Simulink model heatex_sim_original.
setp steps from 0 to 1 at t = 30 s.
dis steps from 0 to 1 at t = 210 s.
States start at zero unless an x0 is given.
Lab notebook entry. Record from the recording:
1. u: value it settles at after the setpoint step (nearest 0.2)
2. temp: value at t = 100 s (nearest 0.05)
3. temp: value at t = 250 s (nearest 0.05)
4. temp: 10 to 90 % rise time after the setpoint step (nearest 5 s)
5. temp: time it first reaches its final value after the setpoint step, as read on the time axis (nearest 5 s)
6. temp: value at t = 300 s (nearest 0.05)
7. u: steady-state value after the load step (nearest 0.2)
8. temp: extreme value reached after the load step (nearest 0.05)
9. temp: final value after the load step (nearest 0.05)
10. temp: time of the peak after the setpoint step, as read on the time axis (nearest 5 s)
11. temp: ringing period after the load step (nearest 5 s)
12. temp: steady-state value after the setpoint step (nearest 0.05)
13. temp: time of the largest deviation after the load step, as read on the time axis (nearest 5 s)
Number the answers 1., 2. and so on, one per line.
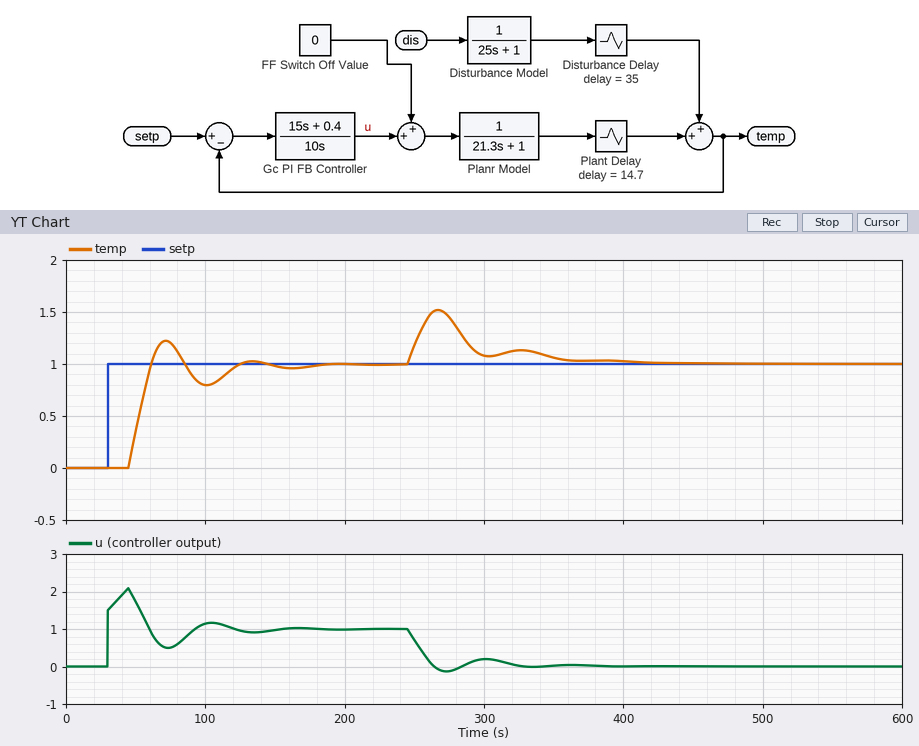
1. 1.0
2. 0.80
3. 1.20
4. 15 s
5. 60 s
6. 1.10
7. 0.0
8. 1.50
9. 1.00
10. 70 s
11. 60 s
12. 1.00
13. 265 s
